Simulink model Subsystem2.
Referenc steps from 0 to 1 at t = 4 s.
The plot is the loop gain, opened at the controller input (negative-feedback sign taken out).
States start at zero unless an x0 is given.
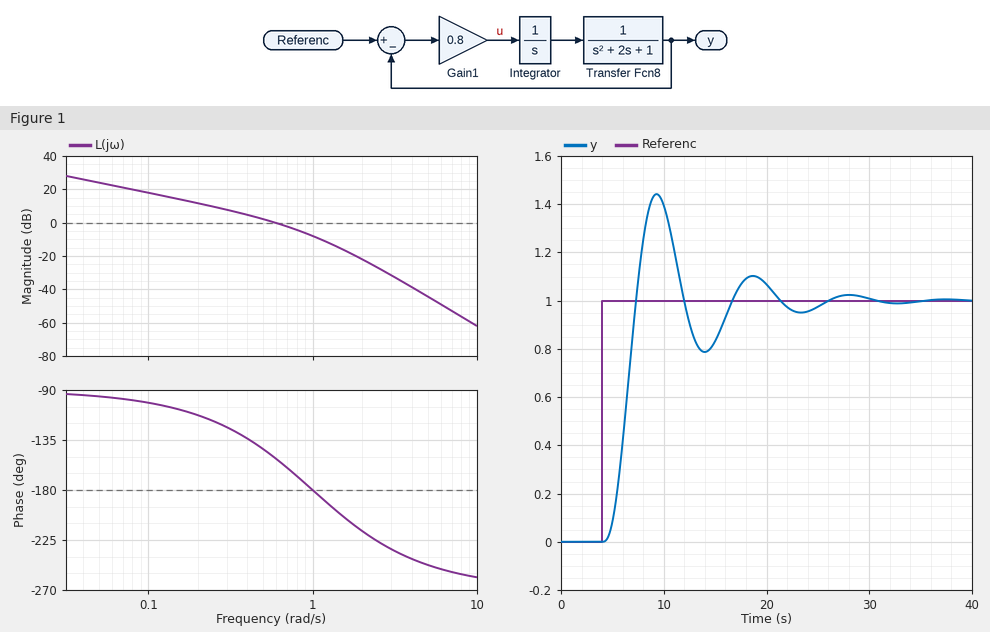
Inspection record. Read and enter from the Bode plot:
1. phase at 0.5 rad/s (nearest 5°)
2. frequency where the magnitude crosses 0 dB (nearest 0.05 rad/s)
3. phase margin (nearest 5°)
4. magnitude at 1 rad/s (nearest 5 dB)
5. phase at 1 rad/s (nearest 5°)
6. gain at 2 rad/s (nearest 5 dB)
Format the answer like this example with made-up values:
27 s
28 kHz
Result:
-145°
0.60 rad/s
30°
-10 dB
-180°
-20 dB
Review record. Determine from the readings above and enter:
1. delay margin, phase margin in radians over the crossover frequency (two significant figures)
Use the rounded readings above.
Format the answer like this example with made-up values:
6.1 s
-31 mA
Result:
0.87 s
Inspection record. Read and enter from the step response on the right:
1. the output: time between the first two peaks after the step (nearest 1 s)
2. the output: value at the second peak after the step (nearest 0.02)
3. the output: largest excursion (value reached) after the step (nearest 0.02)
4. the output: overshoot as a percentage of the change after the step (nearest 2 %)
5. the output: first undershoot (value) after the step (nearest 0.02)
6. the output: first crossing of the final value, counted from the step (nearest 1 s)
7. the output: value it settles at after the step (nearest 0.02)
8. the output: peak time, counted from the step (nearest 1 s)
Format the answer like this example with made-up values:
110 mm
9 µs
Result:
9 s
1.10
1.44
44 %
0.78
3 s
1.00
5 s
